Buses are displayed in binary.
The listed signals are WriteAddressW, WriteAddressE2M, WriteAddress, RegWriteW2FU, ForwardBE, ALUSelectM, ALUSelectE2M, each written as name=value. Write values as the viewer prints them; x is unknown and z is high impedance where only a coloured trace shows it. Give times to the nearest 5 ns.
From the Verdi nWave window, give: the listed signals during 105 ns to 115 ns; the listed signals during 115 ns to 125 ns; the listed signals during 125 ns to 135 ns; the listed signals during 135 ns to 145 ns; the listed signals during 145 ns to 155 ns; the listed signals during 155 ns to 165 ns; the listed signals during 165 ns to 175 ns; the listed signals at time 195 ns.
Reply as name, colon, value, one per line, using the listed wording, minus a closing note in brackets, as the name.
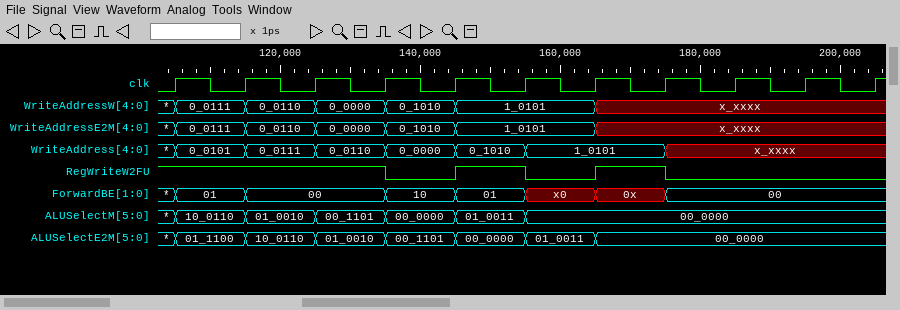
the listed signals during 105 ns to 115 ns: WriteAddressW=0_0111, WriteAddressE2M=0_0111, WriteAddress=0_0101, RegWriteW2FU=1, ForwardBE=01, ALUSelectM=10_0110, ALUSelectE2M=01_1100
the listed signals during 115 ns to 125 ns: WriteAddressW=0_0110, WriteAddressE2M=0_0110, WriteAddress=0_0111, RegWriteW2FU=1, ForwardBE=00, ALUSelectM=01_0010, ALUSelectE2M=10_0110
the listed signals during 125 ns to 135 ns: WriteAddressW=0_0000, WriteAddressE2M=0_0000, WriteAddress=0_0110, RegWriteW2FU=1, ForwardBE=00, ALUSelectM=00_1101, ALUSelectE2M=01_0010
the listed signals during 135 ns to 145 ns: WriteAddressW=0_1010, WriteAddressE2M=0_1010, WriteAddress=0_0000, RegWriteW2FU=0, ForwardBE=10, ALUSelectM=00_0000, ALUSelectE2M=00_1101
the listed signals during 145 ns to 155 ns: WriteAddressW=1_0101, WriteAddressE2M=1_0101, WriteAddress=0_1010, RegWriteW2FU=1, ForwardBE=01, ALUSelectM=01_0011, ALUSelectE2M=00_0000
the listed signals during 155 ns to 165 ns: WriteAddressW=1_0101, WriteAddressE2M=1_0101, WriteAddress=1_0101, RegWriteW2FU=0, ForwardBE=x0, ALUSelectM=00_0000, ALUSelectE2M=01_0011
the listed signals during 165 ns to 175 ns: WriteAddressW=x_xxxx, WriteAddressE2M=x_xxxx, WriteAddress=1_0101, RegWriteW2FU=1, ForwardBE=0x, ALUSelectM=00_0000, ALUSelectE2M=00_0000
the listed signals at time 195 ns: WriteAddressW=x_xxxx, WriteAddressE2M=x_xxxx, WriteAddress=x_xxxx, RegWriteW2FU=0, ForwardBE=00, ALUSelectM=00_0000, ALUSelectE2M=00_0000
